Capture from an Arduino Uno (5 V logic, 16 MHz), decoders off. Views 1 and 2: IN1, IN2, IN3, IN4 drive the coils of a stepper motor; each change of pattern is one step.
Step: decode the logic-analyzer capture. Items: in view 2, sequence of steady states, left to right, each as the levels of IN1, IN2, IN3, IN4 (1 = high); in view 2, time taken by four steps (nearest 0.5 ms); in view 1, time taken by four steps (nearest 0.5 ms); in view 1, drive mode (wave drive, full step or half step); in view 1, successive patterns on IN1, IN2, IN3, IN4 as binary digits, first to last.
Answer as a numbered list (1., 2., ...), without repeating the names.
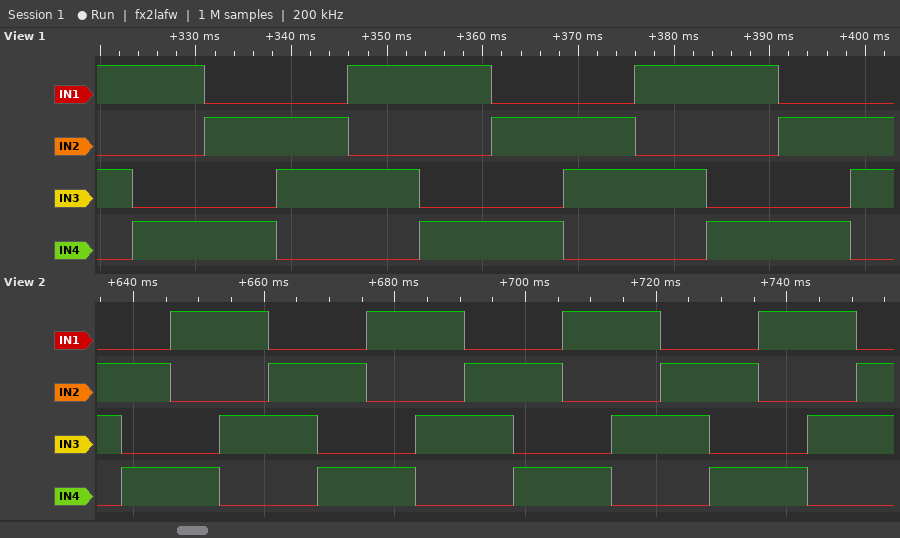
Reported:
1. 0110 0101 1001 1010 0110 0101 1001 1010 0110 0101 1001 1010 0110 0101 1001 1010 0110
2. 30.0 ms
3. 30.0 ms
4. full step
5. 1010 1001 0101 0110 1010 1001 0101 0110 1010 1001 0101 0110
